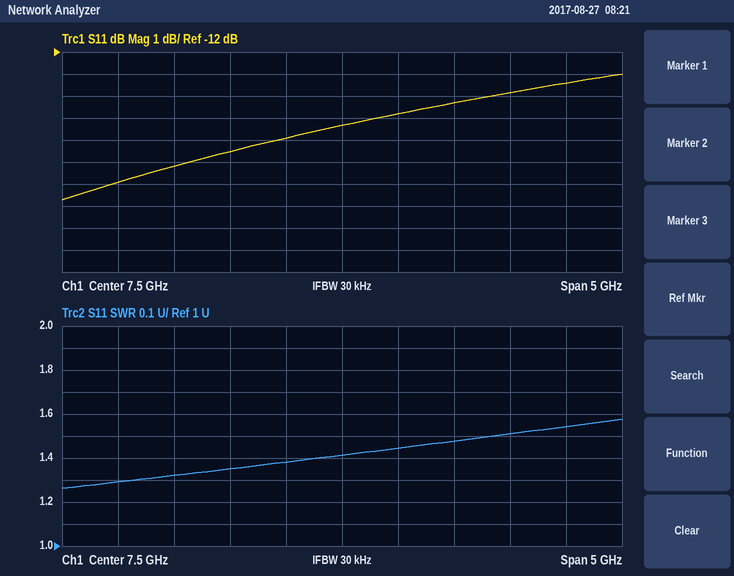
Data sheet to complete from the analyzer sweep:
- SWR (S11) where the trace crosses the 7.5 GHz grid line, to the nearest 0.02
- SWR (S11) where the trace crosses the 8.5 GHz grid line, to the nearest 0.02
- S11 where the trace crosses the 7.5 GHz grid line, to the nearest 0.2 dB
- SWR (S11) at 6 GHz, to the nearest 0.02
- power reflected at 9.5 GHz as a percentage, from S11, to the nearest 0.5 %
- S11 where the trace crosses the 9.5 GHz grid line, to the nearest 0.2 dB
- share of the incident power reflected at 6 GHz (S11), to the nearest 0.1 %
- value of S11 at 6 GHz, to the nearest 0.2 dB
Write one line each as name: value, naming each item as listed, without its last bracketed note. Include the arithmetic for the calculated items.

SWR (S11) where the trace crosses the 7.5 GHz grid line, to the nearest 0.02: 1.42
SWR (S11) where the trace crosses the 8.5 GHz grid line, to the nearest 0.02: 1.48
S11 where the trace crosses the 7.5 GHz grid line, to the nearest 0.2 dB: -15.4 dB
SWR (S11) at 6 GHz, to the nearest 0.02: 1.32
power reflected at 9.5 GHz as a percentage, from S11, to the nearest 0.5 %: 10^(-13.4/10) ≈ 4.57 %, so 4.5 % to the nearest 0.5 %
S11 where the trace crosses the 9.5 GHz grid line, to the nearest 0.2 dB: -13.4 dB
share of the incident power reflected at 6 GHz (S11), to the nearest 0.1 %: 10^(-17.2/10) ≈ 1.9 %
value of S11 at 6 GHz, to the nearest 0.2 dB: -17.2 dB
